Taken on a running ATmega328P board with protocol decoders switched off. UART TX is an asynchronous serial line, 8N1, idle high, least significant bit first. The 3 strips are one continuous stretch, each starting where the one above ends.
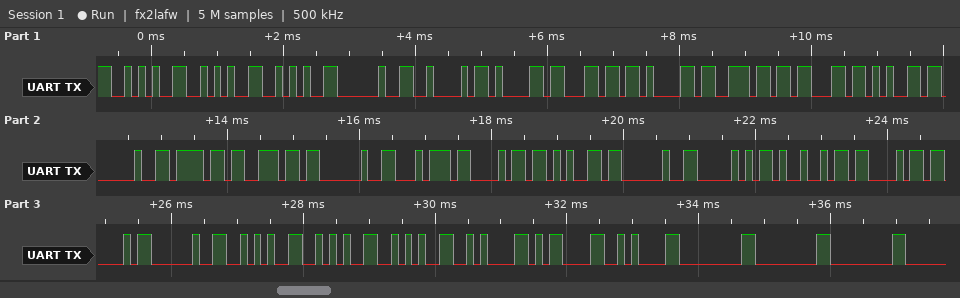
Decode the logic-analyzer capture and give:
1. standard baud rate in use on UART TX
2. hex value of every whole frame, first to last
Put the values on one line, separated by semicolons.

9600 baud; 0x2A 0x2A 0x2A 0x20 0x42 0x61 0x6C 0x61 0x6E 0x63 0x65 0x20 0x6F 0x6E 0x20 0x74 0x68 0x65 0x20 0x50 0x49 0x43 0x43 0x20 0x2A 0x2A 0x2A 0x0A 0x0D 0x0A 0x00 0x00 0x00
